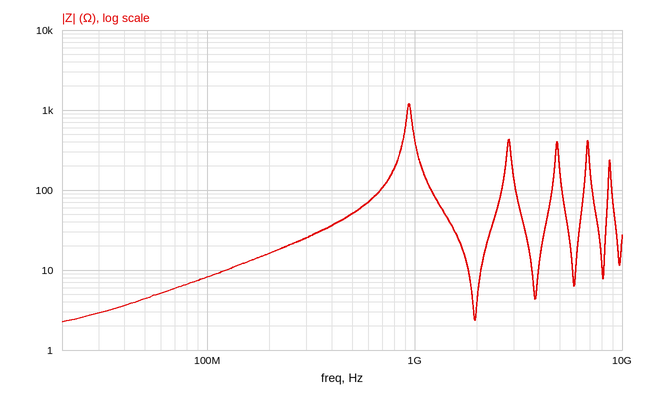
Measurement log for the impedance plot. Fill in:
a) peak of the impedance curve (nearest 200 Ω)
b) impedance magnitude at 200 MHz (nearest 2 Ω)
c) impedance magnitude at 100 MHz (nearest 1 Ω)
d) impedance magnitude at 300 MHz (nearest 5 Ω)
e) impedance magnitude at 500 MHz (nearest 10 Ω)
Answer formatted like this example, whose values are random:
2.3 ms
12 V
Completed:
1.2 kΩ
16 Ω
8 Ω
25 Ω
50 Ω
